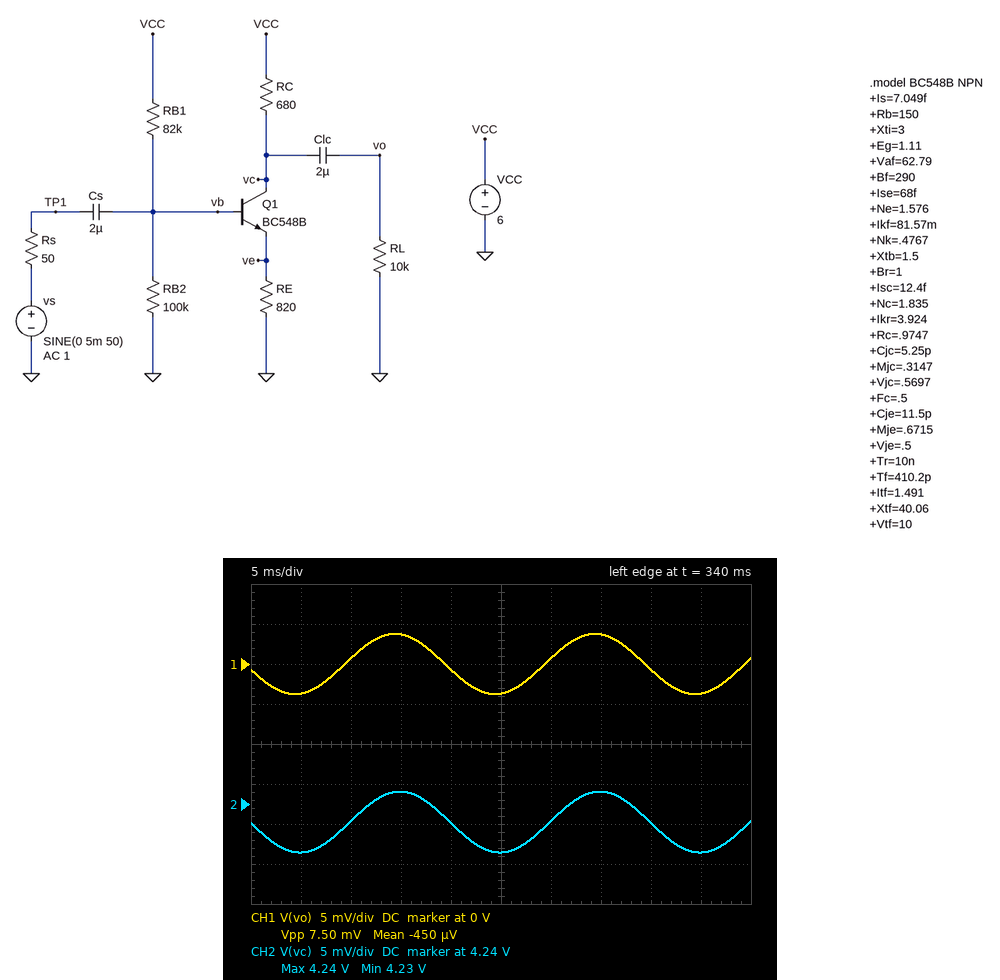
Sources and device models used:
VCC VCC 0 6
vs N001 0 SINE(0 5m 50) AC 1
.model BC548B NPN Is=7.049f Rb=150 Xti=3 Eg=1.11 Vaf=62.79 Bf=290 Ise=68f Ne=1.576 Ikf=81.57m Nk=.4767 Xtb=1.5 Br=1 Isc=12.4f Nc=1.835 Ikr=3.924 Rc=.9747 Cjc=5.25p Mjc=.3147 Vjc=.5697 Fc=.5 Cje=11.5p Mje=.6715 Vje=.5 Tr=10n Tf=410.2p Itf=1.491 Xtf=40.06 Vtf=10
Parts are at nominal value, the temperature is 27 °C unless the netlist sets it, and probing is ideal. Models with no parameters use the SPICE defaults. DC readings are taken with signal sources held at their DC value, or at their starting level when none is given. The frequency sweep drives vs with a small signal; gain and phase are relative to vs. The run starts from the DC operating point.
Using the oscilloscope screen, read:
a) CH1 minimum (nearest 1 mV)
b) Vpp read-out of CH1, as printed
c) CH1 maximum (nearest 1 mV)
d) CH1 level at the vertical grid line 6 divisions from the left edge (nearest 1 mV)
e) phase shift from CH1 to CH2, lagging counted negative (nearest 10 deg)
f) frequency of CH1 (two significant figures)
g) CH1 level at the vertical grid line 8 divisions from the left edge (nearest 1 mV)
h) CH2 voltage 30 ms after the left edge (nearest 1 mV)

-4 mV
7.50 mV
4 mV
1 mV
-10 deg
50 Hz
-1 mV
4.238 V
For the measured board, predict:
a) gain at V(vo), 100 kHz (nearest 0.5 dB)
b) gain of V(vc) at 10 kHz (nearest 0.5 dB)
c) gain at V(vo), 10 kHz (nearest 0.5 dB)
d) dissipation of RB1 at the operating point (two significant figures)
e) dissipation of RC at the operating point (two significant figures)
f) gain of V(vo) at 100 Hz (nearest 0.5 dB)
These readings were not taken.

-2.5 dB
-2.5 dB
-2.5 dB
120 µW
4.6 mW
-2.5 dB
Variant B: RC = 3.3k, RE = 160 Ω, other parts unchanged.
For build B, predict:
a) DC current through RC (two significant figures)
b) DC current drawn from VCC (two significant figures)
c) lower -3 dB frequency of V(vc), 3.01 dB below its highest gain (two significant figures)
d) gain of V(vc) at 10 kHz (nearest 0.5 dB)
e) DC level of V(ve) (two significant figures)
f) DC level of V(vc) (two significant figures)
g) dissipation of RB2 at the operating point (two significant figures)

1.7 mA
1.8 mA
190 Hz
-1.0 dB
280 mV
380 mV
9.4 µW
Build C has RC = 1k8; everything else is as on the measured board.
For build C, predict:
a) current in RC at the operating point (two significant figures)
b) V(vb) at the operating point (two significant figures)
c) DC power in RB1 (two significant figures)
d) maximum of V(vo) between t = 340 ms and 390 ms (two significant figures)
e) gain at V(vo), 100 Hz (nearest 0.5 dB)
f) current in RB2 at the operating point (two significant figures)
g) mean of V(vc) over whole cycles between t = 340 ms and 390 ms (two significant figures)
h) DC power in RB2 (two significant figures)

2.2 mA
2.5 V
150 µW
3.3 mV
-2.5 dB
25 µA
2.0 V
64 µW
